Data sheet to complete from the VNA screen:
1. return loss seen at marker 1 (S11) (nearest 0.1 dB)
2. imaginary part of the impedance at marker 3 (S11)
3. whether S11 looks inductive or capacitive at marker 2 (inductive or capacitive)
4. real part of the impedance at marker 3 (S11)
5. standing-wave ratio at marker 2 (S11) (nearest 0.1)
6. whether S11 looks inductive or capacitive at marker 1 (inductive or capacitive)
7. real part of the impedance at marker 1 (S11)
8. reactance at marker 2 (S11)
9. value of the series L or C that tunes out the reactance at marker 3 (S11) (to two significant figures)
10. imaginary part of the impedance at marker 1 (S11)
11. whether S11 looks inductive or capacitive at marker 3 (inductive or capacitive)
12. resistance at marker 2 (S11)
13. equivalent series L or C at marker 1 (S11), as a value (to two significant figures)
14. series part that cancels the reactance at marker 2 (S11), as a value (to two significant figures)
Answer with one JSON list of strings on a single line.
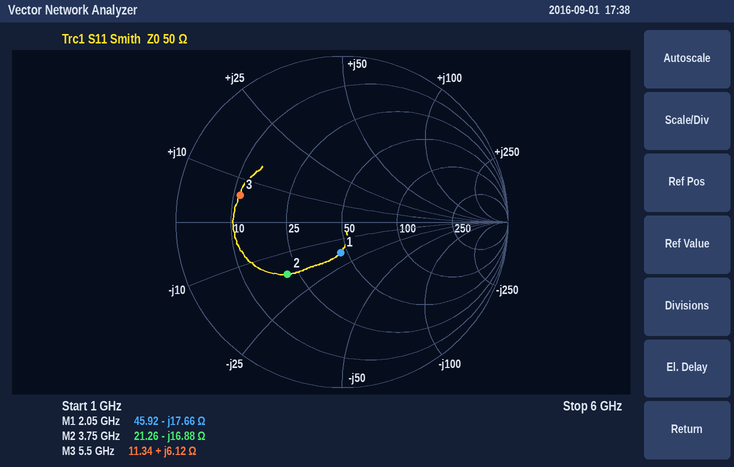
["14.6 dB", "+6.12 Ω", "capacitive", "11.34 Ω", "2.7", "capacitive", "45.92 Ω", "-16.88 Ω", "4.7 pF", "-17.66 Ω", "inductive", "21.26 Ω", "4.4 pF", "720 pH"]
